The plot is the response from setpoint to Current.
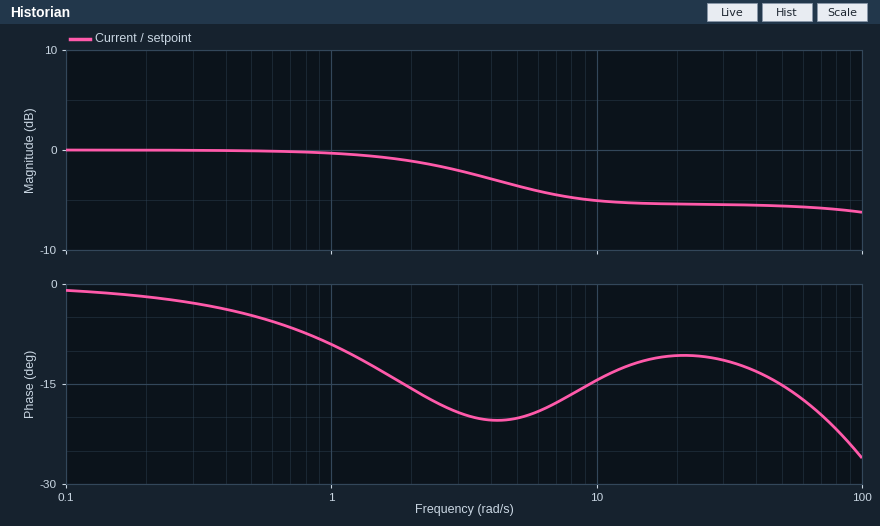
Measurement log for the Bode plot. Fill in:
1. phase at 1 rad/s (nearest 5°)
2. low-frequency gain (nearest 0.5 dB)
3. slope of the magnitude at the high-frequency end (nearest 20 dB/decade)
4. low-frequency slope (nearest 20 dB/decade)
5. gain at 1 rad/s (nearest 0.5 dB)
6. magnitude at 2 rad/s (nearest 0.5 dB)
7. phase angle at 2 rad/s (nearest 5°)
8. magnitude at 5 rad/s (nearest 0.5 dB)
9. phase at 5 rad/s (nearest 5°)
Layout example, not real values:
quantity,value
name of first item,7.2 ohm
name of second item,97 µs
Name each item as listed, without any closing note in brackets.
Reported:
quantity,value
phase at 1 rad/s,-10°
low-frequency gain,0.0 dB
slope of the magnitude at the high-frequency end,0 dB/decade
low-frequency slope,0 dB/decade
gain at 1 rad/s,-0.5 dB
magnitude at 2 rad/s,-1.0 dB
phase angle at 2 rad/s,-15°
magnitude at 5 rad/s,-3.5 dB
phase at 5 rad/s,-20°
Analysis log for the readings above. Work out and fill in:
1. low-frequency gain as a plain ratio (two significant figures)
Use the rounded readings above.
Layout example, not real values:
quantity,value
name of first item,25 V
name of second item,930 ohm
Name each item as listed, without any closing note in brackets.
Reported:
quantity,value
low-frequency gain as a plain ratio,1.0
